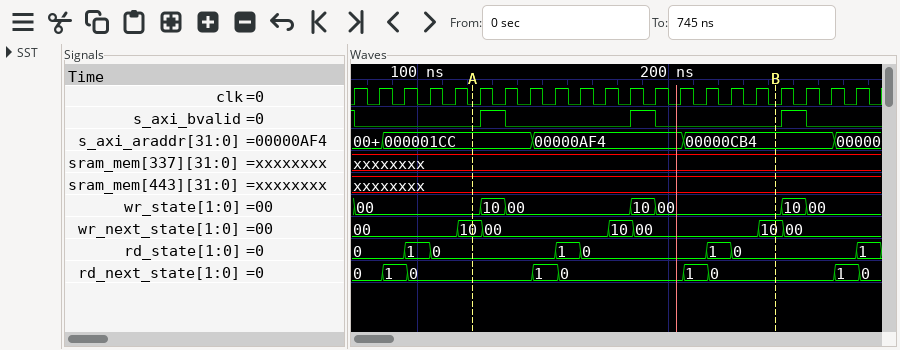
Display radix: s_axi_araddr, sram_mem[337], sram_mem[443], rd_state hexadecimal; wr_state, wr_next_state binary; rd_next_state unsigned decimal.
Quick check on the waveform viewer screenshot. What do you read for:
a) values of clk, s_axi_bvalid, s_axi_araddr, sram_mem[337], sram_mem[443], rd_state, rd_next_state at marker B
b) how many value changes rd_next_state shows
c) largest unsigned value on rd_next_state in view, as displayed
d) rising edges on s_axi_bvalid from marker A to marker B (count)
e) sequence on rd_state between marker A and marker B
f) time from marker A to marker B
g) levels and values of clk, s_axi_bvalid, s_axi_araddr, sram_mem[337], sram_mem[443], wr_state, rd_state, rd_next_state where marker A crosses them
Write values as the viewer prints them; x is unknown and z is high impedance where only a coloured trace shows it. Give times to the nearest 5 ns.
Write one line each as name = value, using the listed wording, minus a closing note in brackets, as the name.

values of clk, s_axi_bvalid, s_axi_araddr, sram_mem[337], sram_mem[443], rd_state, rd_next_state at marker B = clk=0, s_axi_bvalid=0, s_axi_araddr=00000CB4, sram_mem[337]=xxxxxxxx, sram_mem[443]=xxxxxxxx, rd_state=0, rd_next_state=0
how many value changes rd_next_state shows = 8
largest unsigned value on rd_next_state in view, as displayed = 1
rising edges on s_axi_bvalid from marker A to marker B = 2
sequence on rd_state between marker A and marker B = 0, 1, 0, 1, 0
time from marker A to marker B = 120 ns
levels and values of clk, s_axi_bvalid, s_axi_araddr, sram_mem[337], sram_mem[443], wr_state, rd_state, rd_next_state where marker A crosses them = clk=0, s_axi_bvalid=0, s_axi_araddr=000001CC, sram_mem[337]=xxxxxxxx, sram_mem[443]=xxxxxxxx, wr_state=00, rd_state=0, rd_next_state=0
